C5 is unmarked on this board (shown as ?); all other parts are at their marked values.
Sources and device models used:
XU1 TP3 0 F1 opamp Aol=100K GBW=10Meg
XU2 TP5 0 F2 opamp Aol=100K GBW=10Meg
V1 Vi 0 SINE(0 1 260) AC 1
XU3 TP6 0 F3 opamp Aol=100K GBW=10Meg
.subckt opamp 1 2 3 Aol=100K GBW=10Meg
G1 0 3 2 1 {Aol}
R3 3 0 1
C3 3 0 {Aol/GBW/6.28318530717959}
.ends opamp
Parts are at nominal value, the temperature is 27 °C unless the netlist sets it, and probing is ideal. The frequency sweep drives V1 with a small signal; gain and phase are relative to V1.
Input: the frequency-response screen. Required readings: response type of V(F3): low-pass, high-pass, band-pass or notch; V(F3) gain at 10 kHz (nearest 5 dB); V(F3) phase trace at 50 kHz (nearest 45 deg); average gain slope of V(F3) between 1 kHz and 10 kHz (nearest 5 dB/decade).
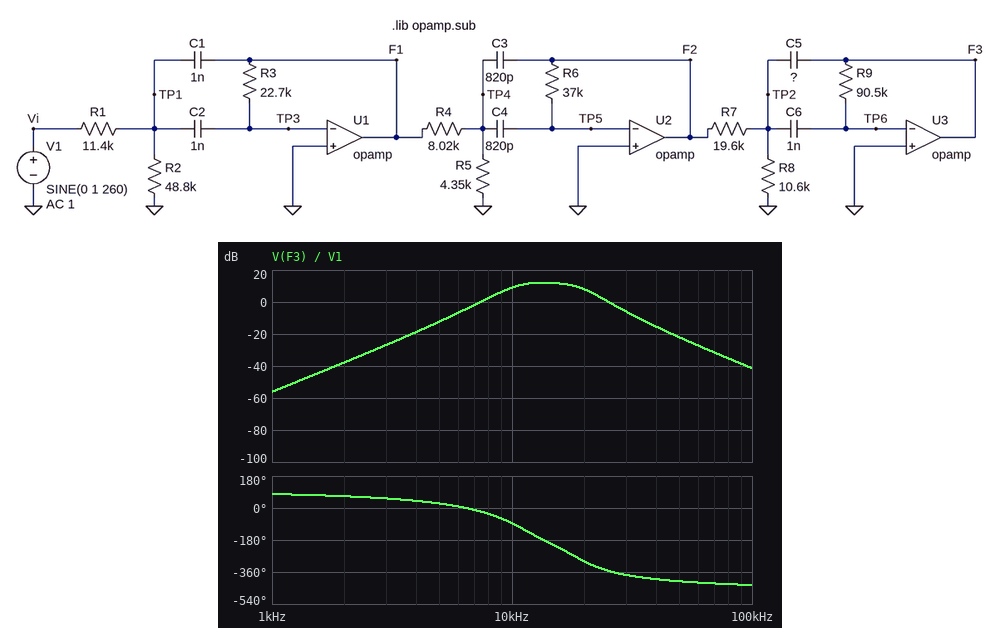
band-pass
10 dB
-405 deg
65 dB/decade
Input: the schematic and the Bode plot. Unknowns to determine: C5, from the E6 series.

330 pF
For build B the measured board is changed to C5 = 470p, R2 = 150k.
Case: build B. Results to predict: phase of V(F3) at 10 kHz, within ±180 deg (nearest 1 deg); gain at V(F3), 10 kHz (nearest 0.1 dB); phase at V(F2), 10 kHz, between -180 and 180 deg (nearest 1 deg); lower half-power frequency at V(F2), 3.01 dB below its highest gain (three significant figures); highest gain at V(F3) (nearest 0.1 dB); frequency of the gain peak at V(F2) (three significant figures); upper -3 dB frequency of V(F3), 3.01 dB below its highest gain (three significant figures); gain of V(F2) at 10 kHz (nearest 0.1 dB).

-124 deg
8.3 dB
70 deg
12.6 kHz
8.6 dB
17.7 kHz
18.7 kHz
-1.3 dB
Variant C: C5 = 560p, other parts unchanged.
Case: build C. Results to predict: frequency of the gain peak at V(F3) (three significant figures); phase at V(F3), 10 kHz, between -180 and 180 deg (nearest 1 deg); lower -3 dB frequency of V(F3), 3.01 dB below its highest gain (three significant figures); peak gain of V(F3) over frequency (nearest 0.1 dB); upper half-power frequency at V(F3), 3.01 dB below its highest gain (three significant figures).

10.5 kHz
-133 deg
7.89 kHz
6.8 dB
18.9 kHz
